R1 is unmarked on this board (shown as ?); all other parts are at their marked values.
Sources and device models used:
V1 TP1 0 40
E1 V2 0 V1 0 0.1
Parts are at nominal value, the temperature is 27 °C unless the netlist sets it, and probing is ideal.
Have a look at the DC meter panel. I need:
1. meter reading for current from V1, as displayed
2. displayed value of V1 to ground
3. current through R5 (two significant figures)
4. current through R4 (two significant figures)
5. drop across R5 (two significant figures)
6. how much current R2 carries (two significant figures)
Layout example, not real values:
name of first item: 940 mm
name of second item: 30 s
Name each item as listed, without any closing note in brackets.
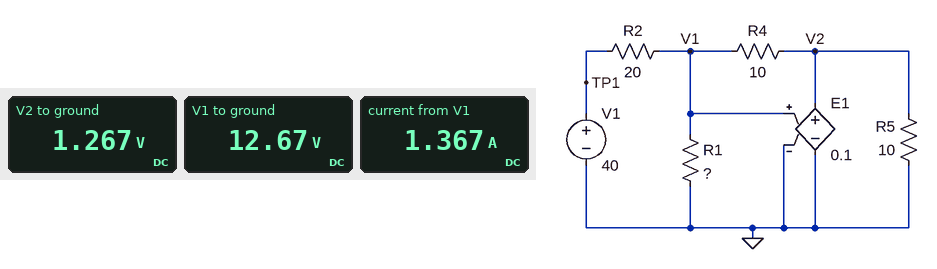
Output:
meter reading for current from V1, as displayed: 1.367 A
displayed value of V1 to ground: 12.67 V
current through R5: 130 mA
current through R4: 1.1 A
drop across R5: 1.3 V
how much current R2 carries: 1.4 A
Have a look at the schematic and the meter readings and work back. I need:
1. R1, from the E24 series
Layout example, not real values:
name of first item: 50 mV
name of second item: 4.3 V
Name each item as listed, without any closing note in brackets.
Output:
R1, from the E24 series: 56 Ω
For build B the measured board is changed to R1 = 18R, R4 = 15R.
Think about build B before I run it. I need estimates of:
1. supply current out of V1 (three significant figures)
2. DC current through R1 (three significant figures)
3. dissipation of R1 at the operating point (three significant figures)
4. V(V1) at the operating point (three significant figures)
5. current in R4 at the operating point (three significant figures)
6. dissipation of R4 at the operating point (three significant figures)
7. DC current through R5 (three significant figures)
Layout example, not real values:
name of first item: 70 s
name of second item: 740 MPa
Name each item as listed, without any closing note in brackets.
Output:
supply current out of V1: 1.40 A
DC current through R1: 671 mA
dissipation of R1 at the operating point: 8.11 W
V(V1) at the operating point: 12.1 V
current in R4 at the operating point: 725 mA
dissipation of R4 at the operating point: 7.88 W
DC current through R5: 121 mA
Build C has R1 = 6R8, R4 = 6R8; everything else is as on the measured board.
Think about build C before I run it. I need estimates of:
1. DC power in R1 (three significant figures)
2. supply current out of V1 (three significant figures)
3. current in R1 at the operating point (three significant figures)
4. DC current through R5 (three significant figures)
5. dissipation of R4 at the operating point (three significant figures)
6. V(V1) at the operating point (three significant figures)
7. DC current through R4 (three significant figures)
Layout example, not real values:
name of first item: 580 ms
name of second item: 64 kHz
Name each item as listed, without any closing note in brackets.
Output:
DC power in R1: 5.42 W
supply current out of V1: 1.70 A
current in R1 at the operating point: 893 mA
DC current through R5: 60.7 mA
dissipation of R4 at the operating point: 4.39 W
V(V1) at the operating point: 6.07 V
DC current through R4: 804 mA
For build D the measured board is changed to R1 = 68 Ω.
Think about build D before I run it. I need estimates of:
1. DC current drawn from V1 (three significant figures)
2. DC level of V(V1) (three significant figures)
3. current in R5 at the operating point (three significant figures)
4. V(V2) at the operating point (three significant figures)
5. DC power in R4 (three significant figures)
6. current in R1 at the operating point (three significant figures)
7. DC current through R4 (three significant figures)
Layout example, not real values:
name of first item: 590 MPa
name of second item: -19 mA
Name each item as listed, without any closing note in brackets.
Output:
DC current drawn from V1: 1.35 A
DC level of V(V1): 12.9 V
current in R5 at the operating point: 129 mA
V(V2) at the operating point: 1.29 V
DC power in R4: 13.5 W
current in R1 at the operating point: 190 mA
DC current through R4: 1.16 A
